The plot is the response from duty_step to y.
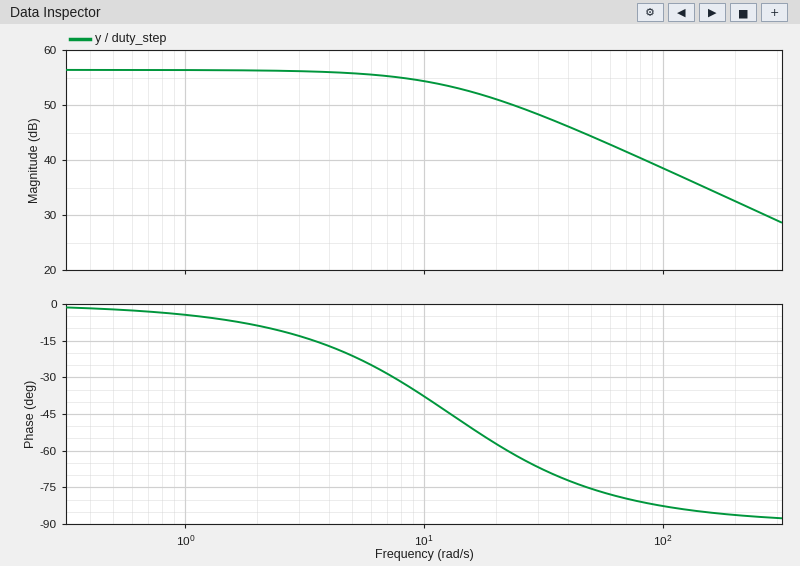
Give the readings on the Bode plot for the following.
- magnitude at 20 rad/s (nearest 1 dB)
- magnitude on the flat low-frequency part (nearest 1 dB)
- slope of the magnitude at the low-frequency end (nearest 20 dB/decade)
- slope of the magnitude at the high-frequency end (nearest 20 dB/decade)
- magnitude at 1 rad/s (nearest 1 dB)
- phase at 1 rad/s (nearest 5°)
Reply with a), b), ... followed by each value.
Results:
a) 51 dB
b) 56 dB
c) 0 dB/decade
d) -20 dB/decade
e) 56 dB
f) -5°
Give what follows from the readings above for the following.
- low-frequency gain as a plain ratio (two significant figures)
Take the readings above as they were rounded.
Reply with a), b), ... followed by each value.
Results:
a) 630
